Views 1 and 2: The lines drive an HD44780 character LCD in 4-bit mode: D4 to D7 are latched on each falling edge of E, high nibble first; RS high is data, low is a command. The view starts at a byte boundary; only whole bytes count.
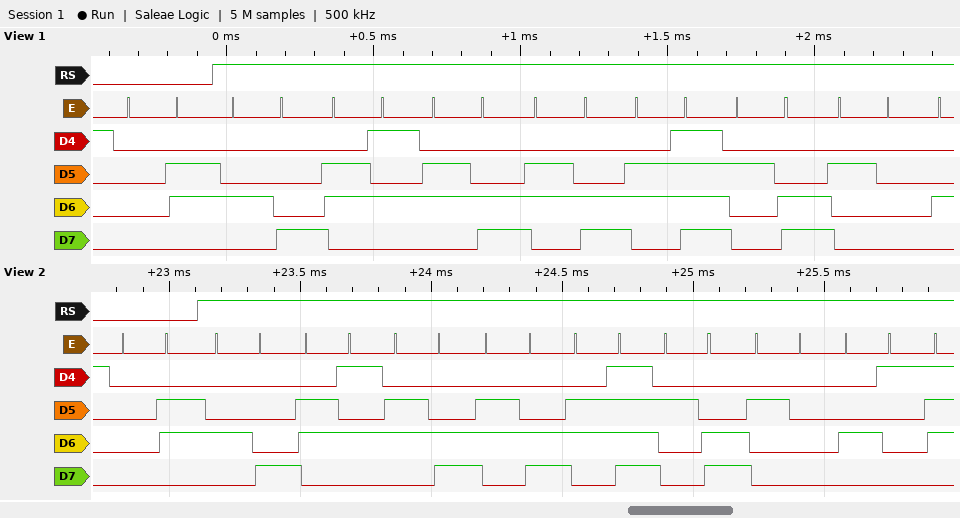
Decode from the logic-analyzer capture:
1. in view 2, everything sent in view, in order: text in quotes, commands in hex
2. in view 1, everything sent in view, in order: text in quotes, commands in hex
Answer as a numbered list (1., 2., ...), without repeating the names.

1. 0x06 "Hello, A"
2. 0x06 "Hello, "
